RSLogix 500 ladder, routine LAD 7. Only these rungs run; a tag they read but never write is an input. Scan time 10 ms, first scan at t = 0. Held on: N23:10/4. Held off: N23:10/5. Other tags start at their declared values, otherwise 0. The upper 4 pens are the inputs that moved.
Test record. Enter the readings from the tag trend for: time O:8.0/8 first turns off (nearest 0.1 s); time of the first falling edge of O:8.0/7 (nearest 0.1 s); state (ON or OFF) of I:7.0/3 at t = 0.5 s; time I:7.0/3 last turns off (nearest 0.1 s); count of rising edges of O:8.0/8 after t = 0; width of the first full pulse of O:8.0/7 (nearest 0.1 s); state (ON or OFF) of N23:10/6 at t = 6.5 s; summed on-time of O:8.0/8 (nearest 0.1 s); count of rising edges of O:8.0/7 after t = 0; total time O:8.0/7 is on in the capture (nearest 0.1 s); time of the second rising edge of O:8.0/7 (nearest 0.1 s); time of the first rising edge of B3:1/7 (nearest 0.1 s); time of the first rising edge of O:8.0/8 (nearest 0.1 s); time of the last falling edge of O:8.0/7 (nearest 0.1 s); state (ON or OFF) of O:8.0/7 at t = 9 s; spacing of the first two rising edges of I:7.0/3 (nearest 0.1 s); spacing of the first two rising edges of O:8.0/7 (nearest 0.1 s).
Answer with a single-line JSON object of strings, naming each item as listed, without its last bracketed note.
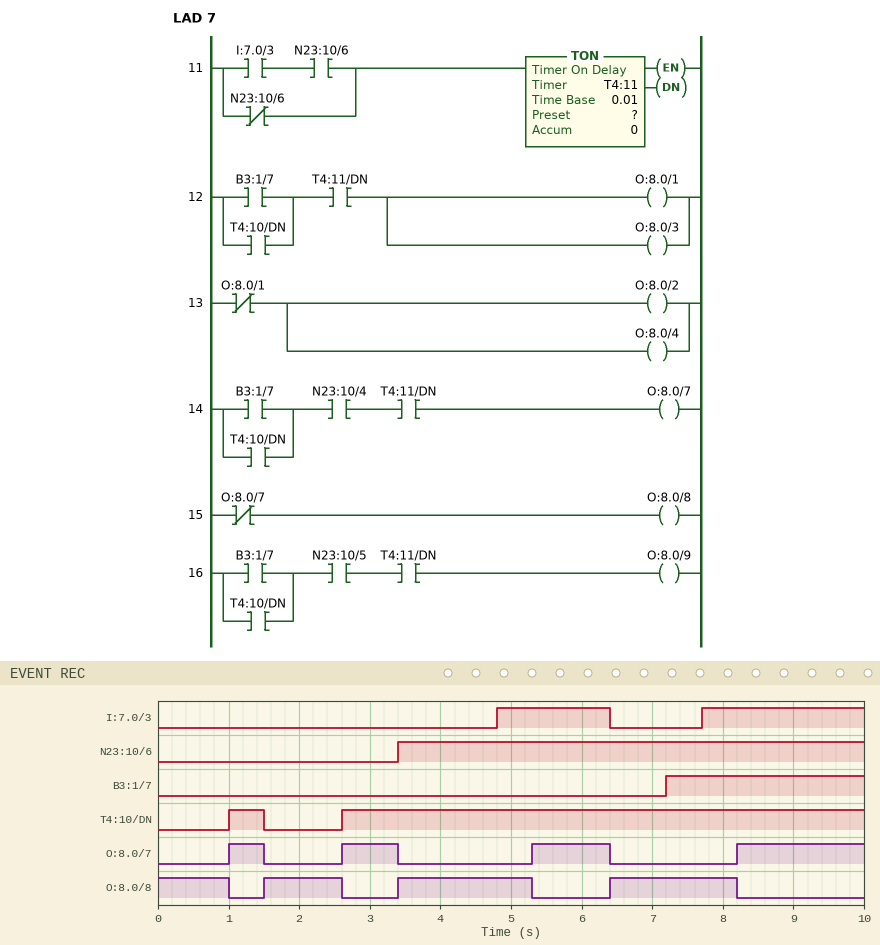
{"time O:8.0/8 first turns off": "1.0 s", "time of the first falling edge of O:8.0/7": "1.5 s", "state (ON or OFF) of I:7.0/3 at t = 0.5 s": "OFF", "time I:7.0/3 last turns off": "6.4 s", "count of rising edges of O:8.0/8 after t = 0": "3", "width of the first full pulse of O:8.0/7": "0.5 s", "state (ON or OFF) of N23:10/6 at t = 6.5 s": "ON", "summed on-time of O:8.0/8": "5.8 s", "count of rising edges of O:8.0/7 after t = 0": "4", "total time O:8.0/7 is on in the capture": "4.2 s", "time of the second rising edge of O:8.0/7": "2.6 s", "time of the first rising edge of B3:1/7": "7.2 s", "time of the first rising edge of O:8.0/8": "1.5 s", "time of the last falling edge of O:8.0/7": "6.4 s", "state (ON or OFF) of O:8.0/7 at t = 9 s": "ON", "spacing of the first two rising edges of I:7.0/3": "2.9 s", "spacing of the first two rising edges of O:8.0/7": "1.6 s"}
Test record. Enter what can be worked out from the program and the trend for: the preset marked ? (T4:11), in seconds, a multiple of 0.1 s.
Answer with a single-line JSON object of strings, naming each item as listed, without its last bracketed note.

{"the preset marked ? (T4:11), in seconds, a multiple of 0.1 s": "0.5 s"}
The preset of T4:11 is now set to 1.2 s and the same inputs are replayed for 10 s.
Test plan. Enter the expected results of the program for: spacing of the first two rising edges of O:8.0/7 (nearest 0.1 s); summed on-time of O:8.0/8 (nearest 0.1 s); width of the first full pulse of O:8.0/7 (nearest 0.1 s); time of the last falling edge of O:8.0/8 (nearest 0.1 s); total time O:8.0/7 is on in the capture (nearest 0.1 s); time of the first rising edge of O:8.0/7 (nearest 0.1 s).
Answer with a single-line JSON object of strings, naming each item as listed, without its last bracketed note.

{"spacing of the first two rising edges of O:8.0/7": "1.4 s", "summed on-time of O:8.0/8": "7.4 s", "width of the first full pulse of O:8.0/7": "0.3 s", "time of the last falling edge of O:8.0/8": "8.9 s", "total time O:8.0/7 is on in the capture": "2.6 s", "time of the first rising edge of O:8.0/7": "1.2 s"}
